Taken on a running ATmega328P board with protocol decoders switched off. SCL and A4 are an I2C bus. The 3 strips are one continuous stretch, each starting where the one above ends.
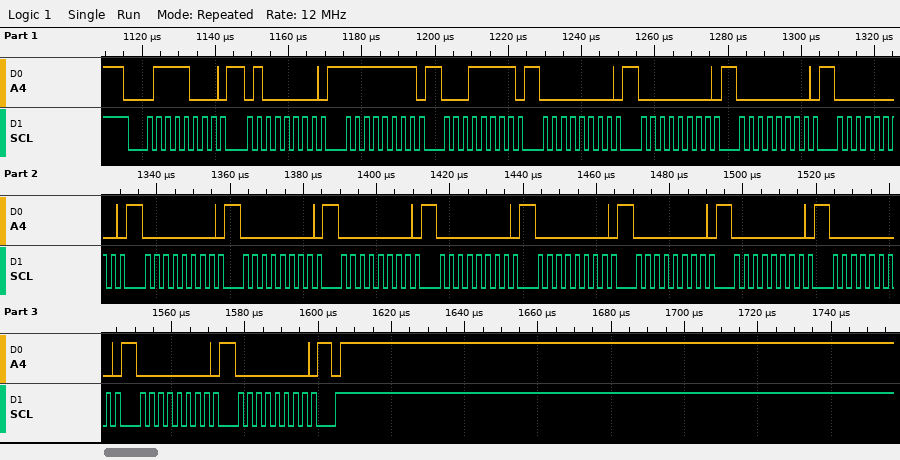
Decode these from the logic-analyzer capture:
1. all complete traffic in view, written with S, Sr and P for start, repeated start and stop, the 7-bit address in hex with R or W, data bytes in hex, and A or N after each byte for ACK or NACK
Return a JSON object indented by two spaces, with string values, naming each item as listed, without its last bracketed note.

{
  "all complete traffic in view, written with S, Sr and P for start, repeated start and stop, the 7-bit address in hex with R or W, data bytes in hex, and A or N after each byte for ACK or NACK": "S 3CW A 40 A FF A 1F A 00 A 00 A 00 A 00 A 00 A 00 A 00 A 00 A 00 A 00 A 00 A 00 A 00 A 00 A P"
}
